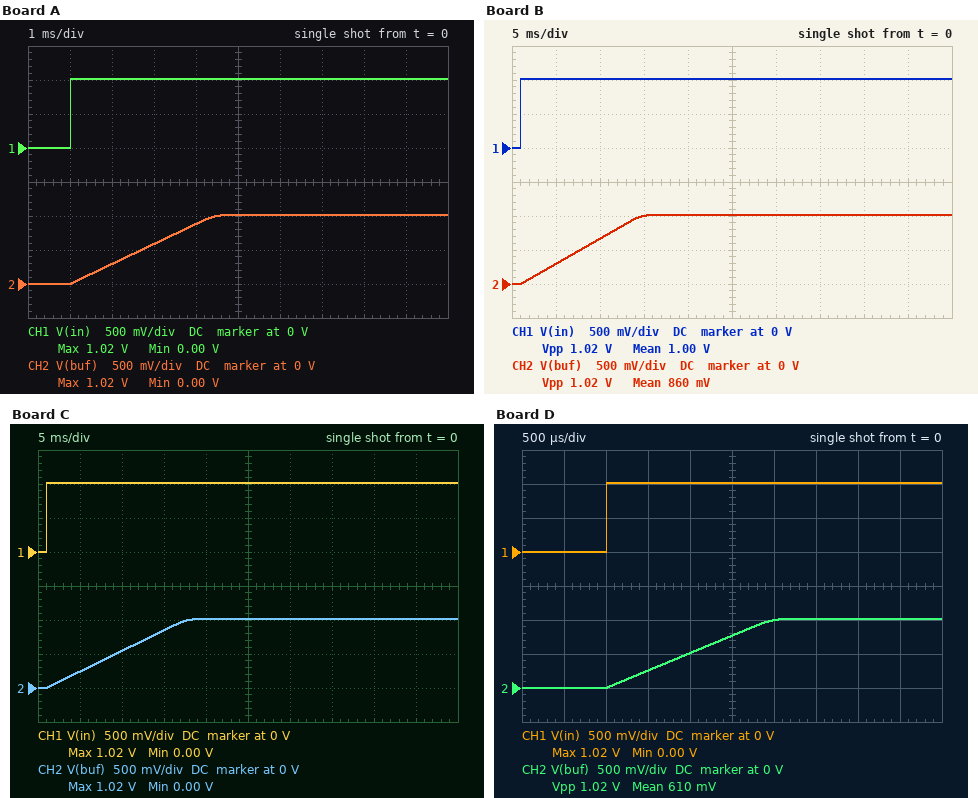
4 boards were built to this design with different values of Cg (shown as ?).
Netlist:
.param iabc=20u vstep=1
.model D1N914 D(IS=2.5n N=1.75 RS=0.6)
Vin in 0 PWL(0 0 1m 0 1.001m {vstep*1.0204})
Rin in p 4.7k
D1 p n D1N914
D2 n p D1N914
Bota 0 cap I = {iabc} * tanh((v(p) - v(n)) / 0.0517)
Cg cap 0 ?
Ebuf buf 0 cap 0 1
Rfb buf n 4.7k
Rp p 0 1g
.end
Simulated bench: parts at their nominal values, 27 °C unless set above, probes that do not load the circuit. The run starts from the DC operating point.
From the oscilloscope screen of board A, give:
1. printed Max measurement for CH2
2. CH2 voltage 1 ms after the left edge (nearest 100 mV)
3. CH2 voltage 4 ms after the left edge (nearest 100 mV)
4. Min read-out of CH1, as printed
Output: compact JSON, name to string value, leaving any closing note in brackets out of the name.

{"printed Max measurement for CH2": "1.02 V", "CH2 voltage 1 ms after the left edge": "0 V", "CH2 voltage 4 ms after the left edge": "900 mV", "Min read-out of CH1, as printed": "0.00 V"}
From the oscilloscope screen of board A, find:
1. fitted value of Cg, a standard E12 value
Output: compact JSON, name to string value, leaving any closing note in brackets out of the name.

{"fitted value of Cg, a standard E12 value": "68 nF"}
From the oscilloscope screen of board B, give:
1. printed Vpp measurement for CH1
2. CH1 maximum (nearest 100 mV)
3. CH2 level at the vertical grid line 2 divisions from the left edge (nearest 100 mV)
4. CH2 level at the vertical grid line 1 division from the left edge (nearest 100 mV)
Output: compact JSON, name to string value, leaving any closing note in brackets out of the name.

{"printed Vpp measurement for CH1": "1.02 V", "CH1 maximum": "1.0 V", "CH2 level at the vertical grid line 2 divisions from the left edge": "700 mV", "CH2 level at the vertical grid line 1 division from the left edge": "300 mV"}
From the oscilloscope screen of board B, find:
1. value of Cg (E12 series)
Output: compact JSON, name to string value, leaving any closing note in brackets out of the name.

{"value of Cg": "270 nF"}
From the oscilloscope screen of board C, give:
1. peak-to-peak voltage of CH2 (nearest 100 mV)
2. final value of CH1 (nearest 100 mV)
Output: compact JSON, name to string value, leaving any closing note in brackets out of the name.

{"peak-to-peak voltage of CH2": "1.0 V", "final value of CH1": "1.0 V"}
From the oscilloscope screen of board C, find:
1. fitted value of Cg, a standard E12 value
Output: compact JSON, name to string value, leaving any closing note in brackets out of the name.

{"fitted value of Cg, a standard E12 value": "330 nF"}
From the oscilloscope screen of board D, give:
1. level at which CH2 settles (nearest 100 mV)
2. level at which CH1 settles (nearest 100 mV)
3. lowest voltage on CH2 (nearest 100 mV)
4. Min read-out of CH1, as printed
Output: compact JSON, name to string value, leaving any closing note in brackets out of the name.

{"level at which CH2 settles": "1.0 V", "level at which CH1 settles": "1.0 V", "lowest voltage on CH2": "0 V", "Min read-out of CH1, as printed": "0.00 V"}
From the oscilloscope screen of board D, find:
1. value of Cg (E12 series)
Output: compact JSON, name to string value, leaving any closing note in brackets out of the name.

{"value of Cg": "39 nF"}
